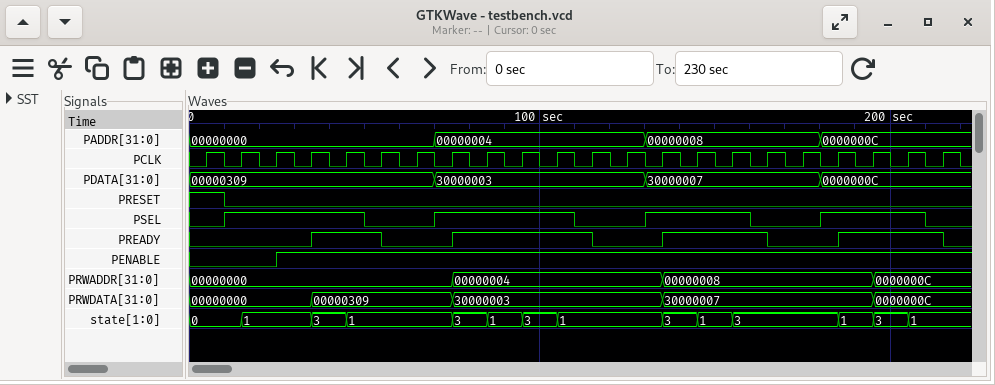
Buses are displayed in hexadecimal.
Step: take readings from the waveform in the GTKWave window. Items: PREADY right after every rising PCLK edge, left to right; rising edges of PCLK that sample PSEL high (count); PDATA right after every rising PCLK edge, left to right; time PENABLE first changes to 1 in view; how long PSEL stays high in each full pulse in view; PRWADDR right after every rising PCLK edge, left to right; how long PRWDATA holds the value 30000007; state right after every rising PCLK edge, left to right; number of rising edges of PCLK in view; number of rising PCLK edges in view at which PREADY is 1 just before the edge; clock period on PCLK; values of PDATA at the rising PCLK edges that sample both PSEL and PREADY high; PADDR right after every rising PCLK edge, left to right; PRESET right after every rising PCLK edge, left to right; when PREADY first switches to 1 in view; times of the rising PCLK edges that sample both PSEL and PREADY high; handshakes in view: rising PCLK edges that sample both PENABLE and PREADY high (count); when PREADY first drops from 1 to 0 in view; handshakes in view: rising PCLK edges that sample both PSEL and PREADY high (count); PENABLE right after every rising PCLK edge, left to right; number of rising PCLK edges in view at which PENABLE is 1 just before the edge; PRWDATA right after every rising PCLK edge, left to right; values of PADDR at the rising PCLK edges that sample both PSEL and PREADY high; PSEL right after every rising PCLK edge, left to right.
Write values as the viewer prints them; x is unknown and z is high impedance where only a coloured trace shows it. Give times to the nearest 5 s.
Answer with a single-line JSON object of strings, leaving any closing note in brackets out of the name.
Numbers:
{"PREADY right after every rising PCLK edge, left to right": "0 0 0 1 1 0 0 1 1 1 1 0 0 1 1 1 0 0 1 1 1 0", "rising edges of PCLK that sample PSEL high": "14", "PDATA right after every rising PCLK edge, left to right": "00000309, 00000309, 00000309, 00000309, 00000309, 00000309, 00000309, 30000003, 30000003, 30000003, 30000003, 30000003, 30000003, 30000007, 30000007, 30000007, 30000007, 30000007, 0000000C, 0000000C, 0000000C, 0000000C", "time PENABLE first changes to 1 in view": "25 s", "how long PSEL stays high in each full pulse in view": "40 s, 40 s, 30 s, 30 s", "PRWADDR right after every rising PCLK edge, left to right": "00000000, 00000000, 00000000, 00000000, 00000000, 00000000, 00000000, 00000004, 00000004, 00000004, 00000004, 00000004, 00000004, 00000008, 00000008, 00000008, 00000008, 00000008, 00000008, 0000000C, 0000000C, 0000000C", "how long PRWDATA holds the value 30000007": "60 s", "state right after every rising PCLK edge, left to right": "0, 1, 1, 3, 1, 1, 1, 3, 1, 3, 1, 1, 1, 3, 1, 3, 3, 3, 1, 3, 1, 1", "number of rising edges of PCLK in view": "22", "number of rising PCLK edges in view at which PREADY is 1 just before the edge": "12", "clock period on PCLK": "10 s", "values of PDATA at the rising PCLK edges that sample both PSEL and PREADY high": "00000309, 30000003, 30000003, 30000003, 30000007, 30000007, 0000000C, 0000000C", "PADDR right after every rising PCLK edge, left to right": "00000000, 00000000, 00000000, 00000000, 00000000, 00000000, 00000000, 00000004, 00000004, 00000004, 00000004, 00000004, 00000004, 00000008, 00000008, 00000008, 00000008, 00000008, 0000000C, 0000000C, 0000000C, 0000000C", "PRESET right after every rising PCLK edge, left to right": "1 0 0 0 0 0 0 0 0 0 0 0 0 0 0 0 0 0 0 0 0 0", "when PREADY first switches to 1 in view": "35 s", "times of the rising PCLK edges that sample both PSEL and PREADY high": "45 s, 85 s, 95 s, 105 s, 145 s, 155 s, 195 s, 205 s", "handshakes in view: rising PCLK edges that sample both PENABLE and PREADY high": "12", "when PREADY first drops from 1 to 0 in view": "55 s", "handshakes in view: rising PCLK edges that sample both PSEL and PREADY high": "8", "PENABLE right after every rising PCLK edge, left to right": "0 0 1 1 1 1 1 1 1 1 1 1 1 1 1 1 1 1 1 1 1 1", "number of rising PCLK edges in view at which PENABLE is 1 just before the edge": "19", "PRWDATA right after every rising PCLK edge, left to right": "00000000, 00000000, 00000000, 00000309, 00000309, 00000309, 00000309, 30000003, 30000003, 30000003, 30000003, 30000003, 30000003, 30000007, 30000007, 30000007, 30000007, 30000007, 30000007, 0000000C, 0000000C, 0000000C", "values of PADDR at the rising PCLK edges that sample both PSEL and PREADY high": "00000000, 00000004, 00000004, 00000004, 00000008, 00000008, 0000000C, 0000000C", "PSEL right after every rising PCLK edge, left to right": "0 1 1 1 1 0 0 1 1 1 1 0 0 1 1 1 0 0 1 1 1 0"}
